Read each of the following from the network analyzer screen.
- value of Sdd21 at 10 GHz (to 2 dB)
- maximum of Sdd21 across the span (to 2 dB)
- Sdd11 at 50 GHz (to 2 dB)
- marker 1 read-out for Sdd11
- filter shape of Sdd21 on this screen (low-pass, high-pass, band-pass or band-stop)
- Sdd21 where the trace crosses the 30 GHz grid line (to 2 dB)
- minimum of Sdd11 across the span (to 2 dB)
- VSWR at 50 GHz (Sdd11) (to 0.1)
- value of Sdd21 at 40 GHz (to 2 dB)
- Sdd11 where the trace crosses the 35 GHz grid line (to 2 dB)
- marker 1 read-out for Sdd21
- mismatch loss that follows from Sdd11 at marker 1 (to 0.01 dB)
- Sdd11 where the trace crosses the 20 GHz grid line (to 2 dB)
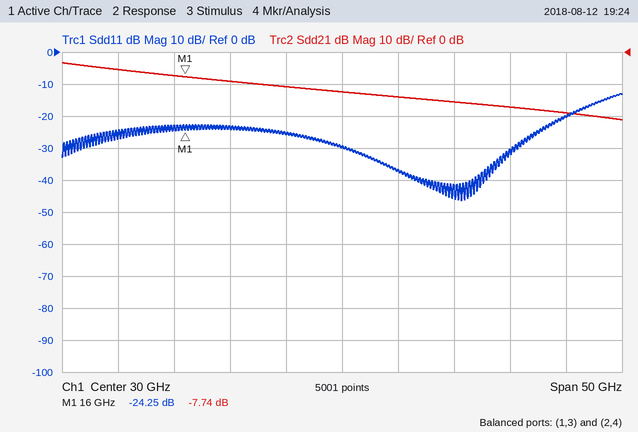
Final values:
-6 dB
-4 dB
-20 dB
-24.25 dB
low-pass
-12 dB
-46 dB
1.2
-16 dB
-36 dB
-7.74 dB
0.02 dB
-24 dB
